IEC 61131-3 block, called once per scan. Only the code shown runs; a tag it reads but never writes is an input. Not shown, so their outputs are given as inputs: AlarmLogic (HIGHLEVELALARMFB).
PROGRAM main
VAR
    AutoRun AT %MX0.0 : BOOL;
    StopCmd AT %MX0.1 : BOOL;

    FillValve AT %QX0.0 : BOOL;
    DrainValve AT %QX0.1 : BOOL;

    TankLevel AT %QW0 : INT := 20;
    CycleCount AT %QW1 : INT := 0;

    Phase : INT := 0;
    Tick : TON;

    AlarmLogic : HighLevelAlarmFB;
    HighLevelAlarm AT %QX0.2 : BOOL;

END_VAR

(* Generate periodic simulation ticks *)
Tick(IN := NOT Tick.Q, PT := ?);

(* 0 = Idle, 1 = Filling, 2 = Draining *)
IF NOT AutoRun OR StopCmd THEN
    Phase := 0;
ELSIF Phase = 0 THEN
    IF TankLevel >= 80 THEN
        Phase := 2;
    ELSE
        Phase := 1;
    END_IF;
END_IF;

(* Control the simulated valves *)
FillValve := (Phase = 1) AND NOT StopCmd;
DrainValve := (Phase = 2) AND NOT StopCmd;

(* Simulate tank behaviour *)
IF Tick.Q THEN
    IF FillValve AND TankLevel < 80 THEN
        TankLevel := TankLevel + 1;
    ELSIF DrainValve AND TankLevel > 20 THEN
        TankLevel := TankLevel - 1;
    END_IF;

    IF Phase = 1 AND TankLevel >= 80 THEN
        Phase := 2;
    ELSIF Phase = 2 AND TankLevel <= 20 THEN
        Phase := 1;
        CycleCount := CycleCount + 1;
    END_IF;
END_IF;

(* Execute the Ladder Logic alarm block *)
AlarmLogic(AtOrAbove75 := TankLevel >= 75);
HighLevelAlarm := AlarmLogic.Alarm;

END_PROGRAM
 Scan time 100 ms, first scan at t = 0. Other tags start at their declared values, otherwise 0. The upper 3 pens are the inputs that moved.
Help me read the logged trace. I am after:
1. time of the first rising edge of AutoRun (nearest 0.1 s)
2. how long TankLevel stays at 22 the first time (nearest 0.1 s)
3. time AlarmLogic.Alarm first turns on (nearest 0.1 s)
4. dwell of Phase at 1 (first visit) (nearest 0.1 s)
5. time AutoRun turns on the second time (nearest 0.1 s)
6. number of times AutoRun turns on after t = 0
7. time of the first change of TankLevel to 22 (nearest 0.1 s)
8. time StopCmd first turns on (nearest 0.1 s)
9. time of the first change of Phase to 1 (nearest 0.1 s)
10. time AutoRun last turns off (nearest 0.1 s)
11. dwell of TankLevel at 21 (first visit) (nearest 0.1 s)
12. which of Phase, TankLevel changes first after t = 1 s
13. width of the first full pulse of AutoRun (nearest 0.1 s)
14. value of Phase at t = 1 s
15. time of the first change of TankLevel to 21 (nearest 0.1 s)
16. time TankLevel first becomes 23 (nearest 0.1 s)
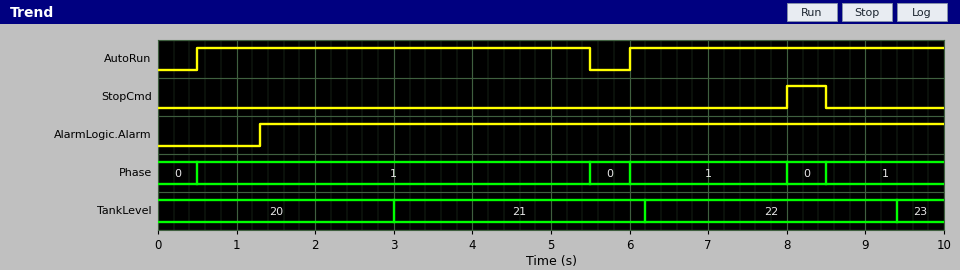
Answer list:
0.5 s
3.2 s
1.3 s
5.0 s
6.0 s
2
6.2 s
8.0 s
0.5 s
5.5 s
3.2 s
TankLevel
5.0 s
1
3.0 s
9.4 s
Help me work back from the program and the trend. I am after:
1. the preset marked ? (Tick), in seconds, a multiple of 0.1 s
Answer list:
3.0 s
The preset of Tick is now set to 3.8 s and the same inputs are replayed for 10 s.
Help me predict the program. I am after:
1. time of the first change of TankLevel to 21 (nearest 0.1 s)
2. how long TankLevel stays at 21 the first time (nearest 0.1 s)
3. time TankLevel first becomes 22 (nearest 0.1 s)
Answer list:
3.8 s
4.0 s
7.8 s
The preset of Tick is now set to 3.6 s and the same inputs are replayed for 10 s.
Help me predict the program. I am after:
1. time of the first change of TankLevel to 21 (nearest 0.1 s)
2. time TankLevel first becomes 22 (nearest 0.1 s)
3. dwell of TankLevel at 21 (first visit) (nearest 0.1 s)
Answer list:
3.6 s
7.4 s
3.8 s
